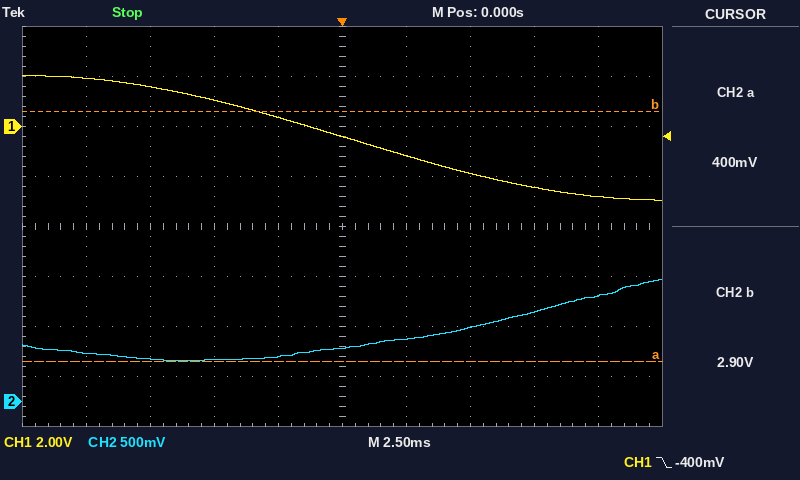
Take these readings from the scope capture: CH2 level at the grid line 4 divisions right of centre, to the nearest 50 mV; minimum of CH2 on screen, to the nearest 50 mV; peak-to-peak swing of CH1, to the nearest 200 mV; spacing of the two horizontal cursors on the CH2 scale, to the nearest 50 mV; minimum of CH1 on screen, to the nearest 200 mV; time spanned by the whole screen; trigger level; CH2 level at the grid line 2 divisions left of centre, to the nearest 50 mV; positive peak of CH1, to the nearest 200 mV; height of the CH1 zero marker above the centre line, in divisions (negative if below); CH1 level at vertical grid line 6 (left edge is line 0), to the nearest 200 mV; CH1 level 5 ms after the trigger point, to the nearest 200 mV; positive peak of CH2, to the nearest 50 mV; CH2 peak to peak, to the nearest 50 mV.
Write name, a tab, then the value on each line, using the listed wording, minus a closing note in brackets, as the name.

CH2 level at the grid line 4 divisions right of centre, to the nearest 50 mV	1.05 V
minimum of CH2 on screen, to the nearest 50 mV	400 mV
peak-to-peak swing of CH1, to the nearest 200 mV	5.0 V
spacing of the two horizontal cursors on the CH2 scale, to the nearest 50 mV	2.50 V
minimum of CH1 on screen, to the nearest 200 mV	-3.0 V
time spanned by the whole screen	25 ms
trigger level	-400 mV
CH2 level at the grid line 2 divisions left of centre, to the nearest 50 mV	400 mV
positive peak of CH1, to the nearest 200 mV	2.0 V
height of the CH1 zero marker above the centre line, in divisions	+2.0 div
CH1 level at vertical grid line 6 (left edge is line 0), to the nearest 200 mV	-1.2 V
CH1 level 5 ms after the trigger point, to the nearest 200 mV	-1.8 V
positive peak of CH2, to the nearest 50 mV	1.20 V
CH2 peak to peak, to the nearest 50 mV	800 mV
